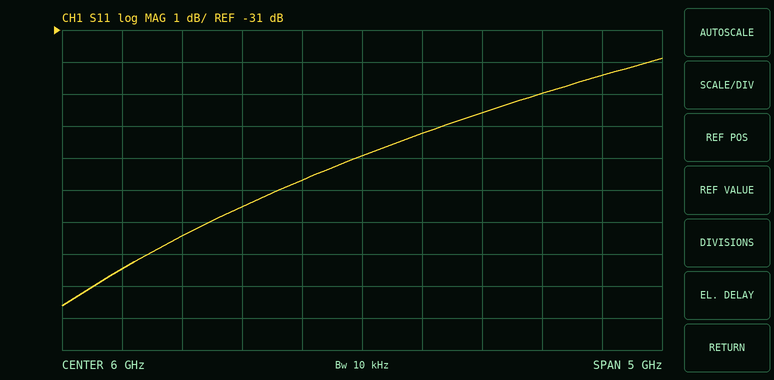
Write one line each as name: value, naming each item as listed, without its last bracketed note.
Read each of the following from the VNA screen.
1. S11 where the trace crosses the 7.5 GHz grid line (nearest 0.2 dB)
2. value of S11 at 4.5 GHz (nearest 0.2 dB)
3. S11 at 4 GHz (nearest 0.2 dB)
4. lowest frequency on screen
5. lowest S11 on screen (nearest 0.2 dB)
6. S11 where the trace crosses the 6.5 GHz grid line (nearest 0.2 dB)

S11 where the trace crosses the 7.5 GHz grid line: -33.0 dB
value of S11 at 4.5 GHz: -37.4 dB
S11 at 4 GHz: -38.4 dB
lowest frequency on screen: 3.5 GHz
lowest S11 on screen: -39.6 dB
S11 where the trace crosses the 6.5 GHz grid line: -34.2 dB
